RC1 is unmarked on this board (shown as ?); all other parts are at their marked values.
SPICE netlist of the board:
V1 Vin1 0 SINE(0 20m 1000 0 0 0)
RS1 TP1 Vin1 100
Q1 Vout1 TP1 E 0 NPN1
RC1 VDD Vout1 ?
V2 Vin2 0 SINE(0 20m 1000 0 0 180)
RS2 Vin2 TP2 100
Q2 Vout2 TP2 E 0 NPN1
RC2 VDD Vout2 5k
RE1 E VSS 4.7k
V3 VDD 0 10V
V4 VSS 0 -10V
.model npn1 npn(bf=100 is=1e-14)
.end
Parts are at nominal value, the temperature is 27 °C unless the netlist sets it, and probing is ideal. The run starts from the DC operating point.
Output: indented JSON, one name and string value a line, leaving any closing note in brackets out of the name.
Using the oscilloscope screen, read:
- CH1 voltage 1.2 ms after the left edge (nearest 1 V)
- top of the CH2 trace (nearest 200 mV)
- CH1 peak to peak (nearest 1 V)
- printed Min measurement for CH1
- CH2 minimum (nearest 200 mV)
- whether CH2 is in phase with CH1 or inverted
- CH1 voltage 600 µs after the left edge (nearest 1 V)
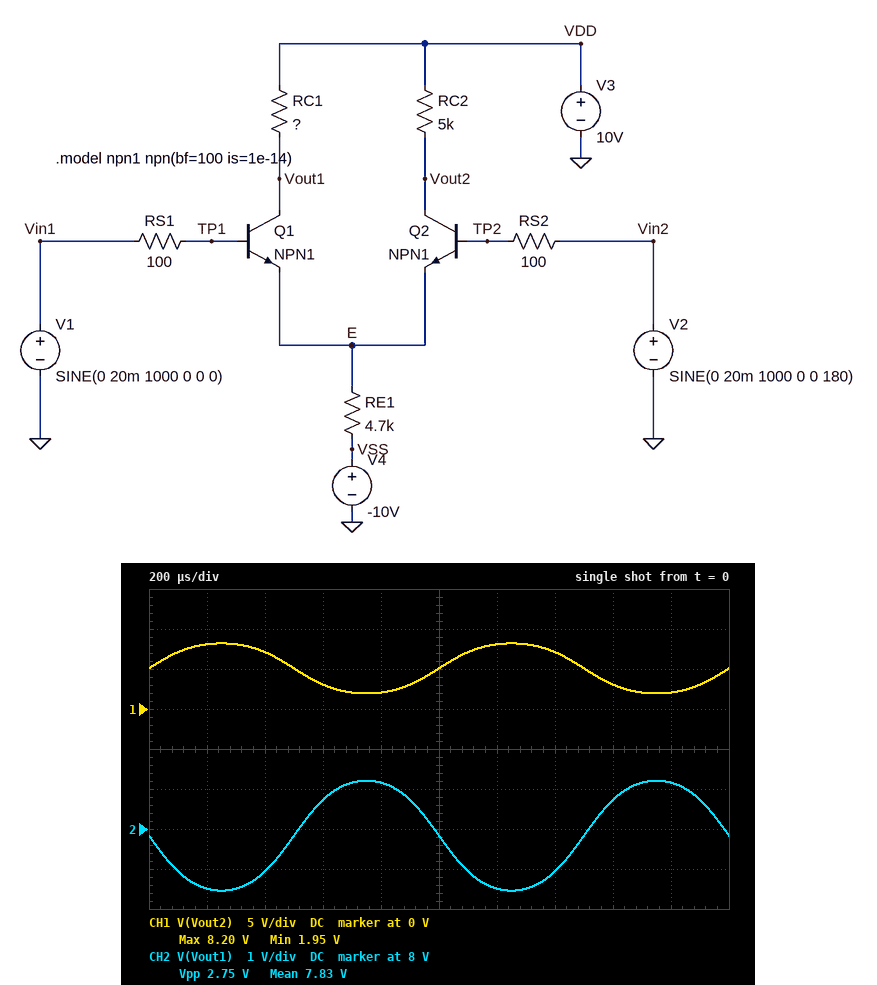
{
  "CH1 voltage 1.2 ms after the left edge": "8 V",
  "top of the CH2 trace": "9.2 V",
  "CH1 peak to peak": "6 V",
  "printed Min measurement for CH1": "1.95 V",
  "CH2 minimum": "6.4 V",
  "whether CH2 is in phase with CH1 or inverted": "inverted",
  "CH1 voltage 600 µs after the left edge": "3 V"
}
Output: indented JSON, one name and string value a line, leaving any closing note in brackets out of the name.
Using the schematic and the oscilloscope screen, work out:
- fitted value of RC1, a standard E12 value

{
  "fitted value of RC1, a standard E12 value": "2.2 kΩ"
}
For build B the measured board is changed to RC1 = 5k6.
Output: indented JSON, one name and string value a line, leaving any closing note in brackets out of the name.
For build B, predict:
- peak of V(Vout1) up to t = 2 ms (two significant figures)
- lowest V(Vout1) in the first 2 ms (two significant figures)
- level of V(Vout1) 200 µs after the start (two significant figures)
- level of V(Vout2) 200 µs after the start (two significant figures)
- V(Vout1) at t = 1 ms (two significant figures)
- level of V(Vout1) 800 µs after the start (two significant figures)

{
  "peak of V(Vout1) up to t = 2 ms": "8.0 V",
  "lowest V(Vout1) in the first 2 ms": "980 mV",
  "level of V(Vout1) 200 µs after the start": "1.1 V",
  "level of V(Vout2) 200 µs after the start": "8.1 V",
  "V(Vout1) at t = 1 ms": "4.5 V",
  "level of V(Vout1) 800 µs after the start": "7.9 V"
}
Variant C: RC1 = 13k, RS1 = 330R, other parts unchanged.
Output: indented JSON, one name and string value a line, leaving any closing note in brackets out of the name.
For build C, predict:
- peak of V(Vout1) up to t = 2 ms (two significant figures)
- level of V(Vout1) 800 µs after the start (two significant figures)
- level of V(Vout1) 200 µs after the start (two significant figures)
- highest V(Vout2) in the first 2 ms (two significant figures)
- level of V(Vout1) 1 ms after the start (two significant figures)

{
  "peak of V(Vout1) up to t = 2 ms": "5.4 V",
  "level of V(Vout1) 800 µs after the start": "5.2 V",
  "level of V(Vout1) 200 µs after the start": "-620 mV",
  "highest V(Vout2) in the first 2 ms": "4.8 V",
  "level of V(Vout1) 1 ms after the start": "-560 mV"
}
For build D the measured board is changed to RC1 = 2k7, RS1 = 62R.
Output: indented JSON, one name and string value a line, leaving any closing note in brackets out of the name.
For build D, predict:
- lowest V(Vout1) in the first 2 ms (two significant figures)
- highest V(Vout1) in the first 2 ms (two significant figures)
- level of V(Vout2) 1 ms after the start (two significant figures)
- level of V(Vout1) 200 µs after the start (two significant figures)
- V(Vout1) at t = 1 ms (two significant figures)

{
  "lowest V(Vout1) in the first 2 ms": "5.6 V",
  "highest V(Vout1) in the first 2 ms": "9.0 V",
  "level of V(Vout2) 1 ms after the start": "5.1 V",
  "level of V(Vout1) 200 µs after the start": "5.7 V",
  "V(Vout1) at t = 1 ms": "7.3 V"
}
